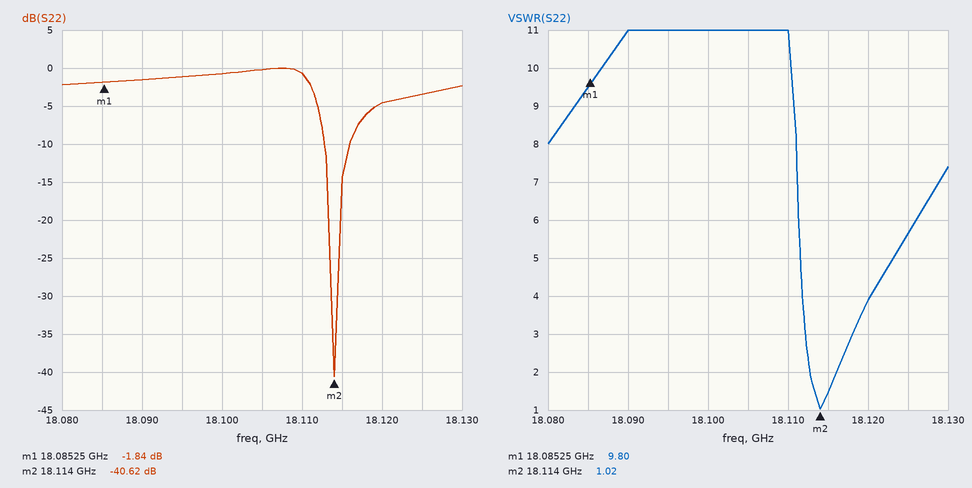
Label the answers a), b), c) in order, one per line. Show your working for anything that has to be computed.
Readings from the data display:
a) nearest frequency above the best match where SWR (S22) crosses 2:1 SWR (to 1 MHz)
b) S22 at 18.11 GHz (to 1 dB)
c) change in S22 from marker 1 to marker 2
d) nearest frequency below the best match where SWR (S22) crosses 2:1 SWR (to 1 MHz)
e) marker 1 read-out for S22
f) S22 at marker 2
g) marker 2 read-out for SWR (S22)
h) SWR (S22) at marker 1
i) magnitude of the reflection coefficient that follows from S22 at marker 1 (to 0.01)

a) 18.116 GHz
b) -1 dB
c) -40.62 − (-1.84) = -38.78 dB
d) 18.113 GHz
e) -1.84 dB
f) -40.62 dB
g) 1.02
h) 9.80
i) 10^(-1.84/20) ≈ 0.81
